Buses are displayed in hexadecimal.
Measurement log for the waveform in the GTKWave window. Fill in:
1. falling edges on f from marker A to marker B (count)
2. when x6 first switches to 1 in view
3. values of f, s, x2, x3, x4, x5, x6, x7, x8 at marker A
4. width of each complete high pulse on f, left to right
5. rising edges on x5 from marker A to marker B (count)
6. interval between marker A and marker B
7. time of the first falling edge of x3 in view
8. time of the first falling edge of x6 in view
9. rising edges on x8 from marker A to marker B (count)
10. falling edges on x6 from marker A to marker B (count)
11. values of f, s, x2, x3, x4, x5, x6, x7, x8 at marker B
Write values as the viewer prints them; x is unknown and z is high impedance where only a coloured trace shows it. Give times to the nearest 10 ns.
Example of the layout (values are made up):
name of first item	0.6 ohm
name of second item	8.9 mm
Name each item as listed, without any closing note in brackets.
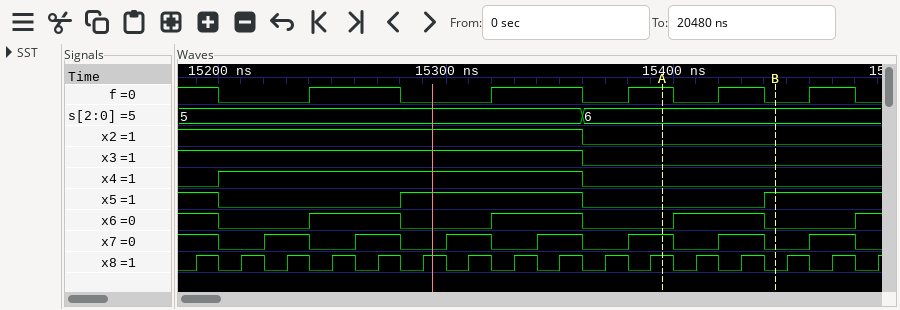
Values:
falling edges on f from marker A to marker B	2
when x6 first switches to 1 in view	15240 ns
values of f, s, x2, x3, x4, x5, x6, x7, x8 at marker A	f=1, s=6, x2=0, x3=0, x4=0, x5=0, x6=0, x7=1, x8=1
width of each complete high pulse on f, left to right	40 ns, 40 ns, 20 ns, 20 ns, 20 ns
rising edges on x5 from marker A to marker B	1
interval between marker A and marker B	50 ns
time of the first falling edge of x3 in view	15360 ns
time of the first falling edge of x6 in view	15200 ns
rising edges on x8 from marker A to marker B	2
falling edges on x6 from marker A to marker B	1
values of f, s, x2, x3, x4, x5, x6, x7, x8 at marker B	f=0, s=6, x2=0, x3=0, x4=0, x5=1, x6=0, x7=0, x8=0
